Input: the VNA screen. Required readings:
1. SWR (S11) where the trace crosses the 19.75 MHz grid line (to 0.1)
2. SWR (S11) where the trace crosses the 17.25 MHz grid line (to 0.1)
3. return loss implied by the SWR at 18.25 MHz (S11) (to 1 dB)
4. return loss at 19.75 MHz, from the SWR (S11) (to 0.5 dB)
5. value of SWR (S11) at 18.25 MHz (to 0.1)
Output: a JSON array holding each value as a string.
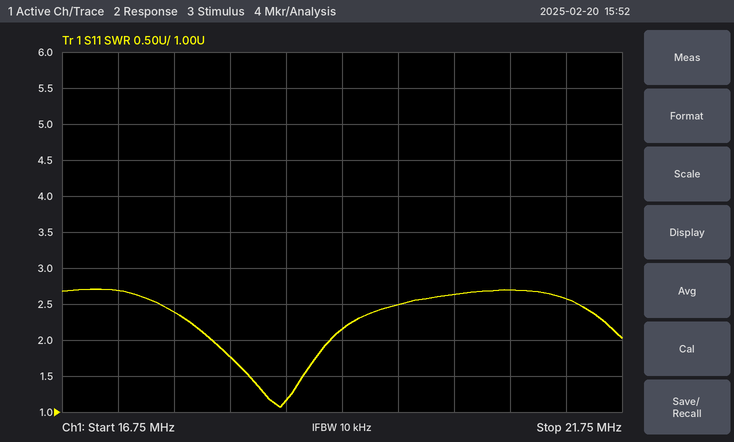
["2.5", "2.7", "11 dB", "7.5 dB", "1.8"]
